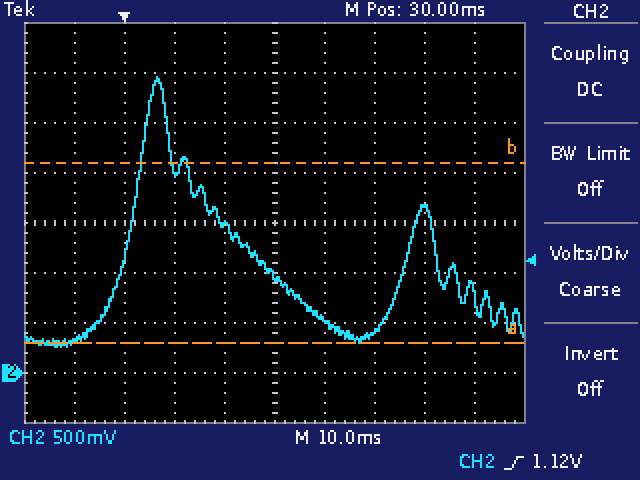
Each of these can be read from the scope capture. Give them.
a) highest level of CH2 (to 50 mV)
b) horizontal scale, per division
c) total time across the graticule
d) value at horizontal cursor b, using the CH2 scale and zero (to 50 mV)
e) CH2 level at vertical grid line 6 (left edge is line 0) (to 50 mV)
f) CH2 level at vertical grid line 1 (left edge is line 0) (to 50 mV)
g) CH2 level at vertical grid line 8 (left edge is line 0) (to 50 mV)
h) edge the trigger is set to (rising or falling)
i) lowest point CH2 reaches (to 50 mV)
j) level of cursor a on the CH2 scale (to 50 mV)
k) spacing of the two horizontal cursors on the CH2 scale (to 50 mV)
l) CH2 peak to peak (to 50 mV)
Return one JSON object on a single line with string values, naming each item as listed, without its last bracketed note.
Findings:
{"highest level of CH2": "2.95 V", "horizontal scale, per division": "10 ms", "total time across the graticule": "100 ms", "value at horizontal cursor b, using the CH2 scale and zero": "2.10 V", "CH2 level at vertical grid line 6 (left edge is line 0)": "550 mV", "CH2 level at vertical grid line 1 (left edge is line 0)": "300 mV", "CH2 level at vertical grid line 8 (left edge is line 0)": "1.65 V", "edge the trigger is set to": "rising", "lowest point CH2 reaches": "250 mV", "level of cursor a on the CH2 scale": "300 mV", "spacing of the two horizontal cursors on the CH2 scale": "1.80 V", "CH2 peak to peak": "2.70 V"}
